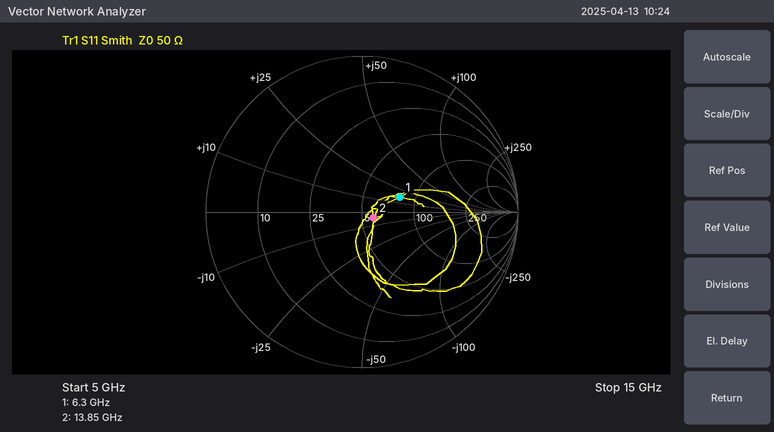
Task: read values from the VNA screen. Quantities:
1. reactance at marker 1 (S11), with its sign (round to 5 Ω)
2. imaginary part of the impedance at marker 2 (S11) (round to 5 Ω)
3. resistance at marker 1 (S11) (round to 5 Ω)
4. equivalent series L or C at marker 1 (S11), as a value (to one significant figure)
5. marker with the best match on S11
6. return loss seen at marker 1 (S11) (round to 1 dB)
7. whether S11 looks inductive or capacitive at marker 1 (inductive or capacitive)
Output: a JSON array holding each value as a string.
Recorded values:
["+15 Ω", "-5 Ω", "80 Ω", "400 pH", "marker 2", "12 dB", "inductive"]
